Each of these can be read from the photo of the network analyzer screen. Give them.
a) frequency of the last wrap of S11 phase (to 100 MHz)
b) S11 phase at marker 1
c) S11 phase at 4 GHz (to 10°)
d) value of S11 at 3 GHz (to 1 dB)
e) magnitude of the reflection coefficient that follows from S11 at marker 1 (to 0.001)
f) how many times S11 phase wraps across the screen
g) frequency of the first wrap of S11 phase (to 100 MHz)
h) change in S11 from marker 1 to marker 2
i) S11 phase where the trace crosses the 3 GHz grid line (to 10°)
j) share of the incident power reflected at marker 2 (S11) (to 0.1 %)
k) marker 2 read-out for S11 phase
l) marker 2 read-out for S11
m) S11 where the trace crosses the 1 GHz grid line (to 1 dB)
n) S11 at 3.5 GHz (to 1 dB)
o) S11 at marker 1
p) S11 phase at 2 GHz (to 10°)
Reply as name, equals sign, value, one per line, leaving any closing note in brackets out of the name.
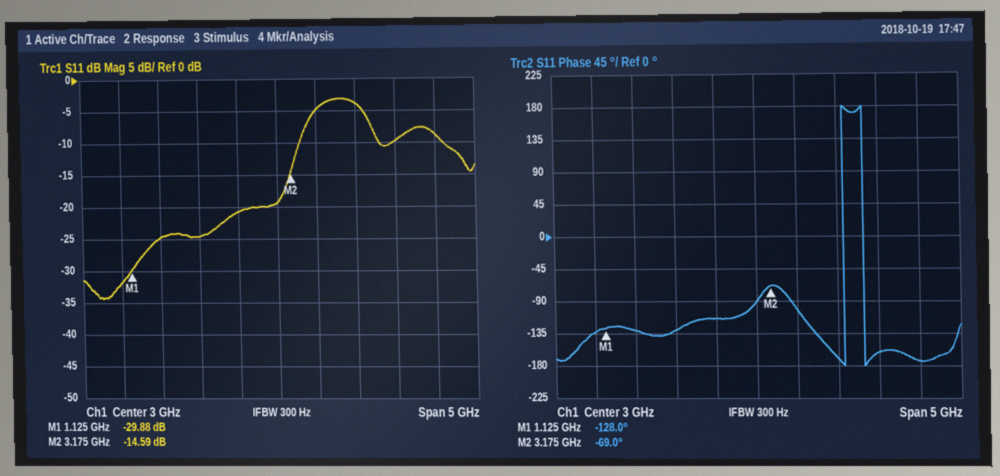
frequency of the last wrap of S11 phase = 4.3 GHz
S11 phase at marker 1 = -128.0°
S11 phase at 4 GHz = -170°
value of S11 at 3 GHz = -19 dB
magnitude of the reflection coefficient that follows from S11 at marker 1 = 0.032
how many times S11 phase wraps across the screen = 2
frequency of the first wrap of S11 phase = 4.1 GHz
change in S11 from marker 1 to marker 2 = 15.29 dB
S11 phase where the trace crosses the 3 GHz grid line = -90°
share of the incident power reflected at marker 2 (S11) = 3.5 %
marker 2 read-out for S11 phase = -69.0°
marker 2 read-out for S11 = -14.59 dB
S11 where the trace crosses the 1 GHz grid line = -32 dB
S11 at 3.5 GHz = -5 dB
S11 at marker 1 = -29.88 dB
S11 phase at 2 GHz = -130°
